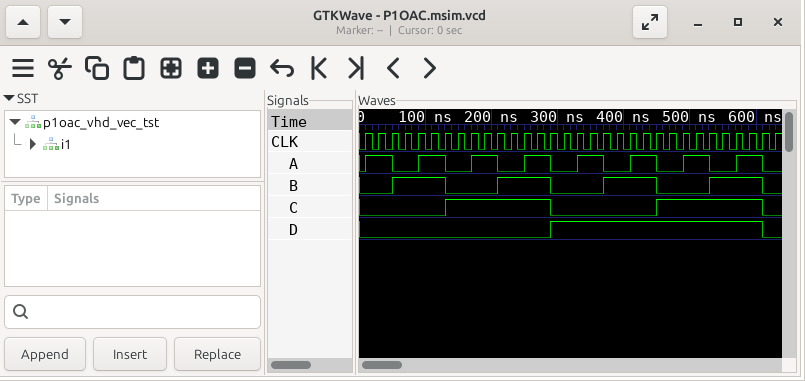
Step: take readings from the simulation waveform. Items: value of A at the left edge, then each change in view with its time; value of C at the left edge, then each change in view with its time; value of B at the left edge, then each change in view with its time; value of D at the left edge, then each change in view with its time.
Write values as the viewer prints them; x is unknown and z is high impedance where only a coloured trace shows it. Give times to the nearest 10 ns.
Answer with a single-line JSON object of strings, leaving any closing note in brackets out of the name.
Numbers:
{"value of A at the left edge, then each change in view with its time": "0, 1 at 10 ns, 0 at 50 ns, 1 at 90 ns, 0 at 130 ns, 1 at 170 ns, 0 at 210 ns, 1 at 250 ns, 0 at 290 ns, 1 at 330 ns, 0 at 370 ns, 1 at 410 ns, 0 at 450 ns, 1 at 490 ns, 0 at 530 ns, 1 at 570 ns, 0 at 610 ns", "value of C at the left edge, then each change in view with its time": "0, 1 at 130 ns, 0 at 290 ns, 1 at 450 ns, 0 at 610 ns", "value of B at the left edge, then each change in view with its time": "0, 1 at 50 ns, 0 at 130 ns, 1 at 210 ns, 0 at 290 ns, 1 at 370 ns, 0 at 450 ns, 1 at 530 ns, 0 at 610 ns", "value of D at the left edge, then each change in view with its time": "0, 1 at 290 ns, 0 at 610 ns"}
